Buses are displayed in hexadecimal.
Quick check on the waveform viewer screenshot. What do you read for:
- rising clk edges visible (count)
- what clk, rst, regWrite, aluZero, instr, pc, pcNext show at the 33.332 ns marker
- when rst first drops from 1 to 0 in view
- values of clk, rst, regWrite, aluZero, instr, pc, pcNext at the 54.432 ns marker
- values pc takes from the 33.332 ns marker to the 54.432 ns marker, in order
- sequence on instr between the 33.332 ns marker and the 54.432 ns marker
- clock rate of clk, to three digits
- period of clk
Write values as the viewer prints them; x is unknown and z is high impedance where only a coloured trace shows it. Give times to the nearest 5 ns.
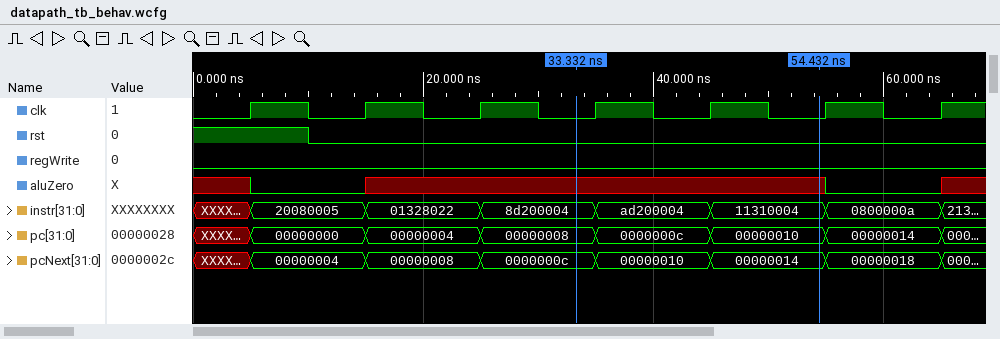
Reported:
7
clk=0, rst=0, regWrite=0, aluZero=x, instr=8d200004, pc=00000008, pcNext=0000000c
10 ns
clk=0, rst=0, regWrite=0, aluZero=x, instr=11310004, pc=00000010, pcNext=00000014
00000008, 0000000c, 00000010
8d200004, ad200004, 11310004
100 MHz
10 ns
